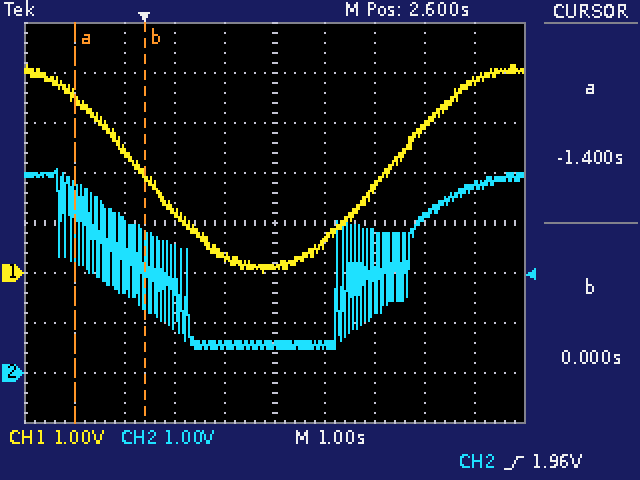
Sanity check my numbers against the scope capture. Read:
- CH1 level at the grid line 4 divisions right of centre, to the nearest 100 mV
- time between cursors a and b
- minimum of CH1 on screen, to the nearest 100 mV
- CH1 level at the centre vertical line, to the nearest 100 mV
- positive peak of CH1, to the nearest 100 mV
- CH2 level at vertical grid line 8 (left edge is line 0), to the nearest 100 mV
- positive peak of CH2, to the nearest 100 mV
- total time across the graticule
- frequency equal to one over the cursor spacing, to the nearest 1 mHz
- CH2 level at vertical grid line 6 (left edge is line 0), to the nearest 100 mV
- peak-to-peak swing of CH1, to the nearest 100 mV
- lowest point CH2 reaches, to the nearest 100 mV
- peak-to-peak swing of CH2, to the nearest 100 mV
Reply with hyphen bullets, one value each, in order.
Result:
- 3.8 V
- 1.4 s
- 0.0 V
- 100 mV
- 4.2 V
- 3.1 V
- 4.1 V
- 10 s
- 714 mHz
- 600 mV
- 4.2 V
- 500 mV
- 3.6 V
